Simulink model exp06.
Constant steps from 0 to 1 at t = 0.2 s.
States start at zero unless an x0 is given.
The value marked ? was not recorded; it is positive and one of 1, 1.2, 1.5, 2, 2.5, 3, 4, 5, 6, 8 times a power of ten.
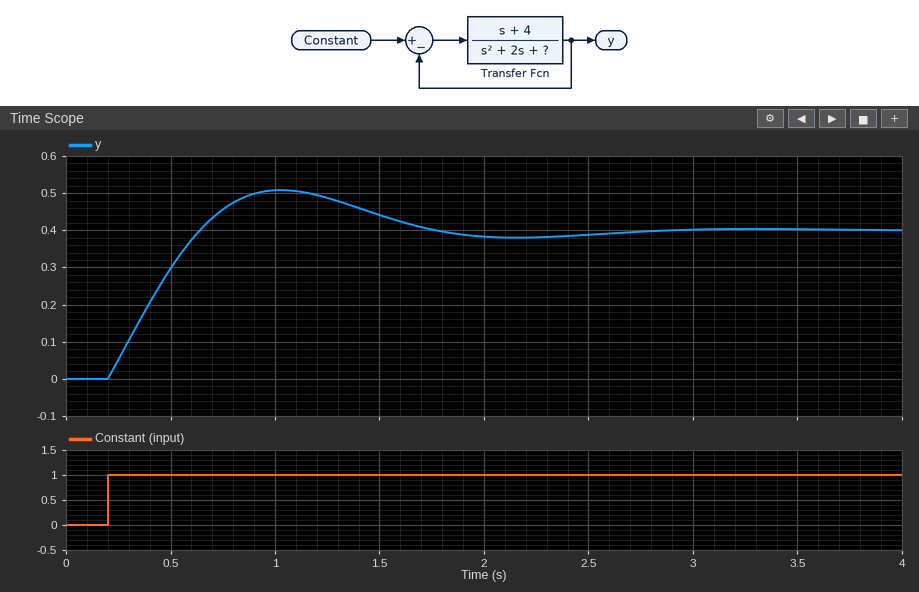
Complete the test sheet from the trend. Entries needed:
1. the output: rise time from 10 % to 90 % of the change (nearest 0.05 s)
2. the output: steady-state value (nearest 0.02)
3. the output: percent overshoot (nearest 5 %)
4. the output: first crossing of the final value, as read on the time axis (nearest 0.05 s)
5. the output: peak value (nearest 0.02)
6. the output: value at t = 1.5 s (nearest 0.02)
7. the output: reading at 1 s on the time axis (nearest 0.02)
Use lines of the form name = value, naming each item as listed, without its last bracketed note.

the output: rise time from 10 % to 90 % of the change = 0.35 s
the output: steady-state value = 0.40
the output: percent overshoot = 25 %
the output: first crossing of the final value, as read on the time axis = 0.65 s
the output: peak value = 0.50
the output: value at t = 1.5 s = 0.44
the output: reading at 1 s on the time axis = 0.50
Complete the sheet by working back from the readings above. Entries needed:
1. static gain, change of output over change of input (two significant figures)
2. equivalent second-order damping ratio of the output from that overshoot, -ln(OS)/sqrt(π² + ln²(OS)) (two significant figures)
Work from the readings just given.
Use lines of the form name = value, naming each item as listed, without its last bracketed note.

static gain, change of output over change of input = 0.40
equivalent second-order damping ratio of the output from that overshoot, -ln(OS)/sqrt(π² + ln²(OS)) = 0.40
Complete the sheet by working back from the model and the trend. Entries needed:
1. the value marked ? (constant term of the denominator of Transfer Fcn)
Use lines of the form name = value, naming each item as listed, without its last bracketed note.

the value marked ? = 6
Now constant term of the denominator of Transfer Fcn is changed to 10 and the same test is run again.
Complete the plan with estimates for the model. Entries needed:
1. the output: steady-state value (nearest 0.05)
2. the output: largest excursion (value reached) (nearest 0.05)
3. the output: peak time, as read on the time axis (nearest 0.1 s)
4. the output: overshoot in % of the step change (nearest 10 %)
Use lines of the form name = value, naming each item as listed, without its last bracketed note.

the output: steady-state value = 0.30
the output: largest excursion (value reached) = 0.40
the output: peak time, as read on the time axis = 0.8 s
the output: overshoot in % of the step change = 40 %
